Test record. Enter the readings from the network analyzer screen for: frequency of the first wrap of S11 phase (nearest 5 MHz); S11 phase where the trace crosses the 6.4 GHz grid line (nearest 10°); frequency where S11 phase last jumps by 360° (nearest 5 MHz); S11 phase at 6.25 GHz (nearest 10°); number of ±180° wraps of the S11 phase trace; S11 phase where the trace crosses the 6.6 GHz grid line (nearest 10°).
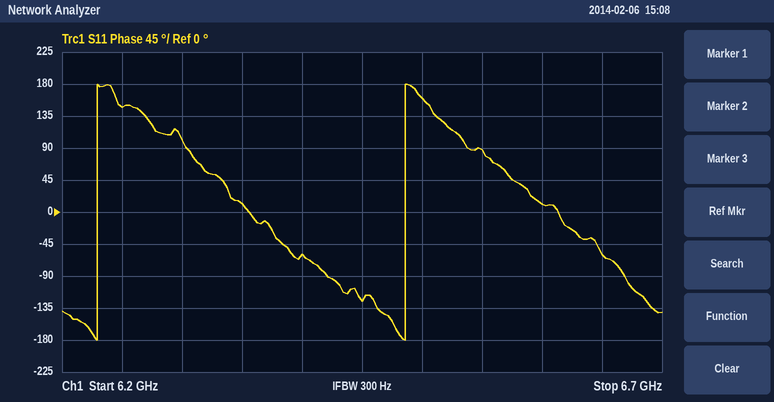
6.230 GHz
-60°
6.485 GHz
150°
2
10°
